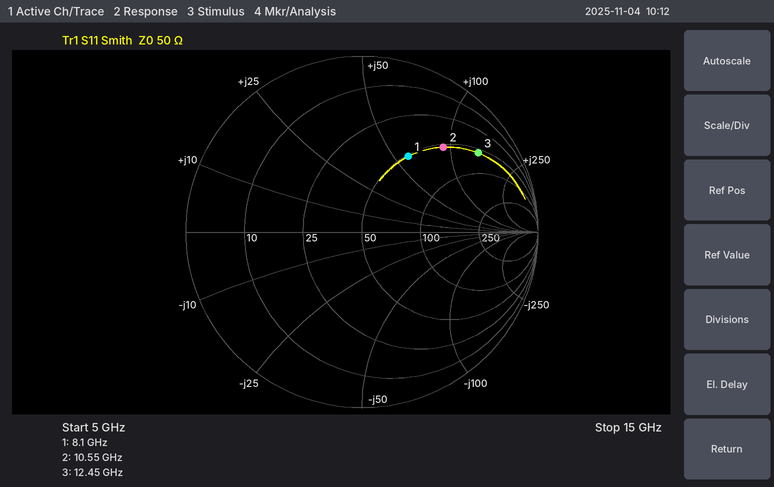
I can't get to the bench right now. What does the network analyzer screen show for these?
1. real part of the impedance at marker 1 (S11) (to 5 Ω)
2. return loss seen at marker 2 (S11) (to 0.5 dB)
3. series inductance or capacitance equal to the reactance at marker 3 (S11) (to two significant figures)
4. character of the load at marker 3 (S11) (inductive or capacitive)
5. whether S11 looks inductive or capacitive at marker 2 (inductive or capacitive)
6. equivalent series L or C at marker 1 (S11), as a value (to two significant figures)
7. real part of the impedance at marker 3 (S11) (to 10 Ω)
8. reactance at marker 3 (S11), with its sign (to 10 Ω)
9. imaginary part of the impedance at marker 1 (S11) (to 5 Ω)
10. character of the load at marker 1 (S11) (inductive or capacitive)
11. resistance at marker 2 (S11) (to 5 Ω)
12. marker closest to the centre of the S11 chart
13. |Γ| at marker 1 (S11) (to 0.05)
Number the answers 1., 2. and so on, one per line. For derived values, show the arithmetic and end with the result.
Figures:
1. 50 Ω
2. 3.5 dB
3. L = 140 Ω/(2π × 12.45 GHz) ≈ 1.8 nH
4. inductive
5. inductive
6. L = 60 Ω/(2π × 8.1 GHz) ≈ 1.2 nH
7. 60 Ω
8. +140 Ω
9. +60 Ω
10. inductive
11. 55 Ω
12. marker 1
13. 0.50
